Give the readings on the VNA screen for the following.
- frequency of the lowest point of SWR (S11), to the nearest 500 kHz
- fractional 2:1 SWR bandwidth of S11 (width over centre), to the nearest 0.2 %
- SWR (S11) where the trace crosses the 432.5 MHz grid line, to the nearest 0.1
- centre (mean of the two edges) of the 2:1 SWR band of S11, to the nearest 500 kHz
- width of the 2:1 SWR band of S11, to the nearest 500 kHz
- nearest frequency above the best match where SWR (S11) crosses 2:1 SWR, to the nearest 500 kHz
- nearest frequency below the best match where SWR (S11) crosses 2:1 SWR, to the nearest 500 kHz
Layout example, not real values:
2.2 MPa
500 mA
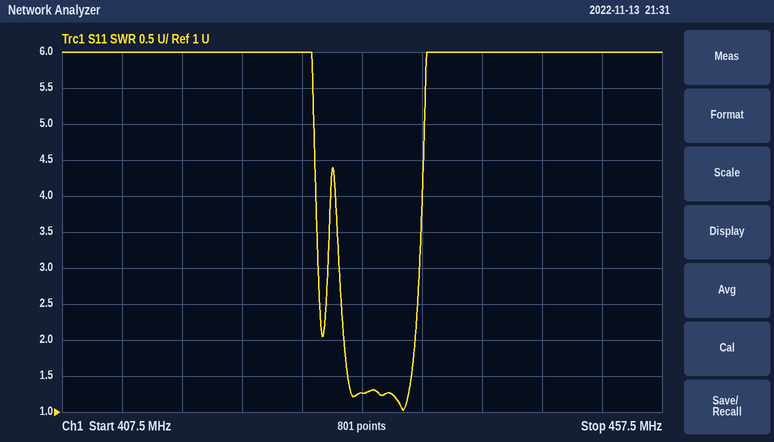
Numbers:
436.0 MHz
1.4 %
1.3
434.0 MHz
6.0 MHz
437.0 MHz
431.0 MHz
